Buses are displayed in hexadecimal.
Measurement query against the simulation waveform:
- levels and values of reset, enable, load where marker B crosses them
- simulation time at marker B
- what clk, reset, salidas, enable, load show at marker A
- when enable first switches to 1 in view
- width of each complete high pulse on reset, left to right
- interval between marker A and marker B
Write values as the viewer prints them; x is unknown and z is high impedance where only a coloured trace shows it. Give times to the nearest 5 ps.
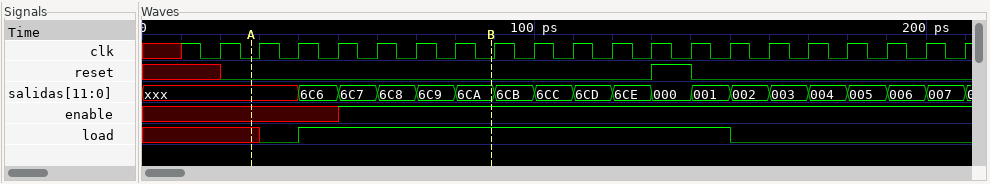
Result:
reset=0, enable=1, load=1
90 ps
clk=0, reset=0, salidas=xxx, enable=x, load=x
50 ps
10 ps
60 ps
